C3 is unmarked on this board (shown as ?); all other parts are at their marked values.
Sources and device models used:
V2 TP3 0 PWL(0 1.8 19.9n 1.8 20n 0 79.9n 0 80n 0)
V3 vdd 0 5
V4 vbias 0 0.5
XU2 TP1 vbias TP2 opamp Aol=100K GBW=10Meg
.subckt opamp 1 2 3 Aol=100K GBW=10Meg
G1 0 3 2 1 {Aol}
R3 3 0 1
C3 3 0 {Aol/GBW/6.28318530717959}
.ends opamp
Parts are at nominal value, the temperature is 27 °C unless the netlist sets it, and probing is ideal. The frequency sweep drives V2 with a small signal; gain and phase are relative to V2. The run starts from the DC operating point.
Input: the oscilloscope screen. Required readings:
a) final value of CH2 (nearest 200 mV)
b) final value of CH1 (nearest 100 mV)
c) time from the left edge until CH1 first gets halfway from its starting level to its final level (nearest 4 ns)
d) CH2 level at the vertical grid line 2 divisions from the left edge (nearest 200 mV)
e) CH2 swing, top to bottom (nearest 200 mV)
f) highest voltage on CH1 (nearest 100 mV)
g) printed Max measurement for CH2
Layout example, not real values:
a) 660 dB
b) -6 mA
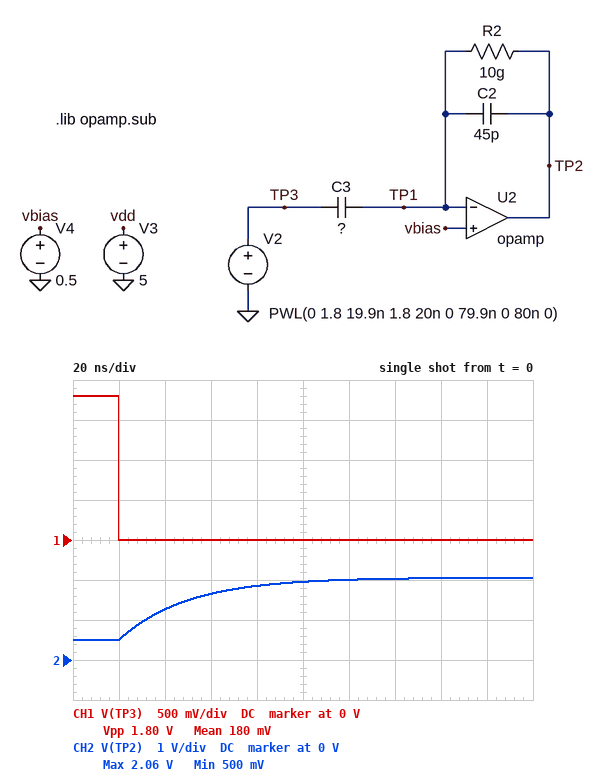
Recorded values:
a) 2.0 V
b) 0 V
c) 20 ns
d) 1.2 V
e) 1.6 V
f) 1.8 V
g) 2.06 V
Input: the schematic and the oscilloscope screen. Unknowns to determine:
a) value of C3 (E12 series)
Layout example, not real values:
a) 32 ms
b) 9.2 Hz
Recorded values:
a) 39 pF
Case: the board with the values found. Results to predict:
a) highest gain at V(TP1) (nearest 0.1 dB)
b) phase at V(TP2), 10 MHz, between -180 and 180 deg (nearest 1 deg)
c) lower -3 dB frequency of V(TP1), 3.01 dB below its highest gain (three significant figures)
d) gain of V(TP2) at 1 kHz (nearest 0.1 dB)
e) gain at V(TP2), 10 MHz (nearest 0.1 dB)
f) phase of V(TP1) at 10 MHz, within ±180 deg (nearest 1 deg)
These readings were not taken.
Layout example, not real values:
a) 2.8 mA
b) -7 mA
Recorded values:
a) -6.7 dB
b) 118 deg
c) 5.36 MHz
d) -1.2 dB
e) -7.8 dB
f) 28 deg
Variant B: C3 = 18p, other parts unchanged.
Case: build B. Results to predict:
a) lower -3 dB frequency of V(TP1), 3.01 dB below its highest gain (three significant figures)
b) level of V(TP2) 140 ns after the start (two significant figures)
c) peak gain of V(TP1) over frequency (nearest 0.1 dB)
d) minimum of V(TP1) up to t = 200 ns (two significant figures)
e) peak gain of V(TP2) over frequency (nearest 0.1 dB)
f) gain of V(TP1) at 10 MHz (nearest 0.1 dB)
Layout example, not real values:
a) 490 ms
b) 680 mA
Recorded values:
a) 7.14 MHz
b) 1.2 V
c) -10.9 dB
d) -13 mV
e) -8.0 dB
f) -12.7 dB
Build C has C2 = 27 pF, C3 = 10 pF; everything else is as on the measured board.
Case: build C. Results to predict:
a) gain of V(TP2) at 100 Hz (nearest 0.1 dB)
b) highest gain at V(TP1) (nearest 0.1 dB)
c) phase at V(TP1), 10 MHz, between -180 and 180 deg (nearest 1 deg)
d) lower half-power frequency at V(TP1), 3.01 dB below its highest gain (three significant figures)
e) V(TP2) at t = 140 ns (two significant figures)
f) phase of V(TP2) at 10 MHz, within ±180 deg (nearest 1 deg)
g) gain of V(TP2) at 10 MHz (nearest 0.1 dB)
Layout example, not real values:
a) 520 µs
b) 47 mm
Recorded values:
a) -8.6 dB
b) -11.4 dB
c) 36 deg
d) 7.30 MHz
e) 1.2 V
f) 126 deg
g) -13.2 dB
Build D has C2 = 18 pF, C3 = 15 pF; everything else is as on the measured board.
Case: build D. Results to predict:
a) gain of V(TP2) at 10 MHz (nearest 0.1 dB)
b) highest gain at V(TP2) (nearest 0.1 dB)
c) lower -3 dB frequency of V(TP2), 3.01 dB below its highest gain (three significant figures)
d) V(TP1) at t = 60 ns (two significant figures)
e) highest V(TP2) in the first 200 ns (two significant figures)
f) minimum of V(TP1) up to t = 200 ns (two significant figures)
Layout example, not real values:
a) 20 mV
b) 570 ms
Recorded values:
a) -8.0 dB
b) -1.6 dB
c) 884 mHz
d) 290 mV
e) 2.0 V
f) -320 mV
